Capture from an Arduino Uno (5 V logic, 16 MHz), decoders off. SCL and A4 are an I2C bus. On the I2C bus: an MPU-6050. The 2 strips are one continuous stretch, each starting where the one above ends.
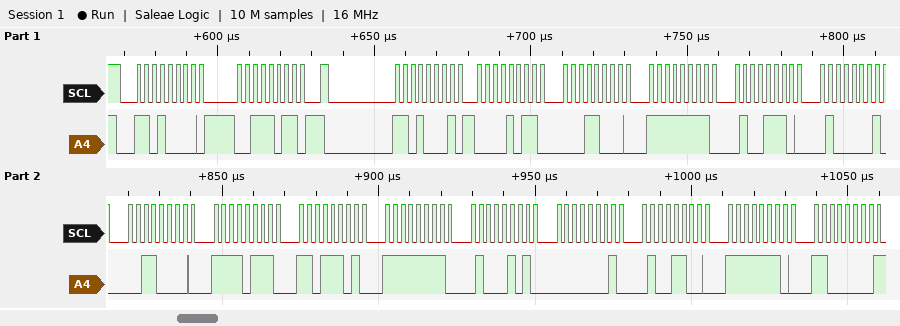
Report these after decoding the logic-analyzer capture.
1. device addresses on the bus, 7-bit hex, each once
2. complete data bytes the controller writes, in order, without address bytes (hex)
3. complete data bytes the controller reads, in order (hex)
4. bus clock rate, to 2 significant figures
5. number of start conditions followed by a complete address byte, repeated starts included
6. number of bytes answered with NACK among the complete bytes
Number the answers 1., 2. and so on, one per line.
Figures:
1. 0x68
2. 3B
3. 0B 18 FF 4E 41 30 F7 DD FF 45 01 4C FE C0
4. 400 kHz
5. 2
6. 1
